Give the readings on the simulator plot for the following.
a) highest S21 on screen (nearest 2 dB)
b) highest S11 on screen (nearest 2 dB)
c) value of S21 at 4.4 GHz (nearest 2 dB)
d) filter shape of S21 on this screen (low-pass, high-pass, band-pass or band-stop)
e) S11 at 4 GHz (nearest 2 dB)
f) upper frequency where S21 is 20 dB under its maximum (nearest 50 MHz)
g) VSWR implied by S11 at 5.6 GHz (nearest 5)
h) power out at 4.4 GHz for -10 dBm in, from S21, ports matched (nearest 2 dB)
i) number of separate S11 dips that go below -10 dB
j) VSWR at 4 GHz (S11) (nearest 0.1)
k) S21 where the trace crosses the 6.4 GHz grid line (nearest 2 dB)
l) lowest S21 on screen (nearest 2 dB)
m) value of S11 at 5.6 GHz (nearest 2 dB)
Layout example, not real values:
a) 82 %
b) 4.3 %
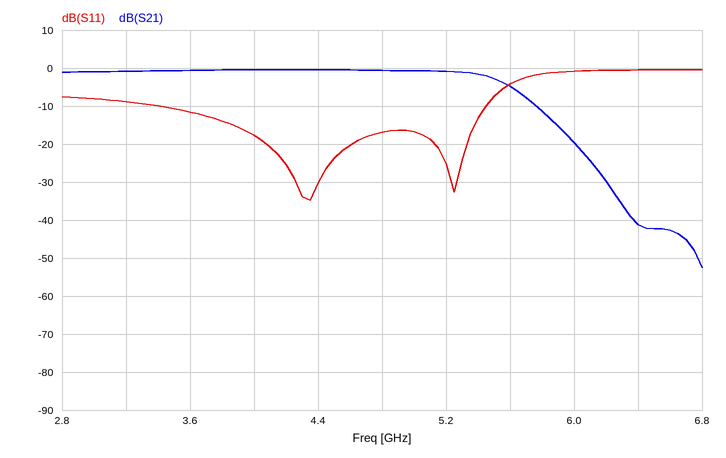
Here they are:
a) 0 dB
b) 0 dB
c) 0 dB
d) low-pass
e) -18 dB
f) 6.00 GHz
g) 5
h) -10 dBm
i) 2
j) 1.3
k) -42 dB
l) -52 dB
m) -4 dB
